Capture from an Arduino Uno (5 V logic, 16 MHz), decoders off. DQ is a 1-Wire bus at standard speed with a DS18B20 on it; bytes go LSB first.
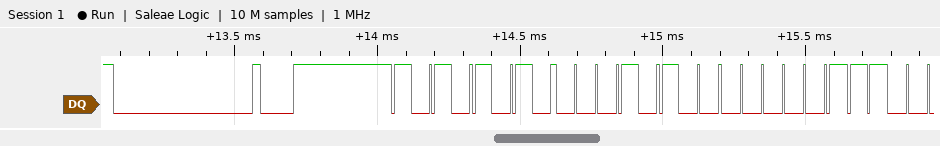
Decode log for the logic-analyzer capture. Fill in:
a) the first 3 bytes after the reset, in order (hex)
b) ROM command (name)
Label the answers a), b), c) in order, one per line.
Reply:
a) 55 28 E0
b) Match ROM
